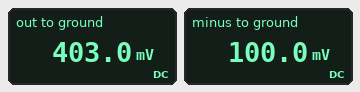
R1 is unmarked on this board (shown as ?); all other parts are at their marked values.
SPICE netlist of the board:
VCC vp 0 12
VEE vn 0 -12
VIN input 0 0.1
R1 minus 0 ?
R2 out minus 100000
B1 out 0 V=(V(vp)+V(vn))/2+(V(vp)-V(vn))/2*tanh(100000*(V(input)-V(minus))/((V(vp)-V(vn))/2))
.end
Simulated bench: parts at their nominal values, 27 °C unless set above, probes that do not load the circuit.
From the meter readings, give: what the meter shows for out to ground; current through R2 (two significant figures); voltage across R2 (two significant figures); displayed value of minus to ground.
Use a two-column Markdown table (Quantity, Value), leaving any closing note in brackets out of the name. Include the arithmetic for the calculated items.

| Quantity | Value |
|---|---|
| what the meter shows for out to ground | 403.0 mV |
| current through R2 | (403 mV - 100 mV) / 100 kΩ = 3.0 µA |
| voltage across R2 | 403 mV - 100 mV = 300 mV |
| displayed value of minus to ground | 100.0 mV |
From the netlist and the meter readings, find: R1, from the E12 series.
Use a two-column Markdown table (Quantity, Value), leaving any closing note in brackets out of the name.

| Quantity | Value |
|---|---|
| R1, from the E12 series | 33 kΩ |
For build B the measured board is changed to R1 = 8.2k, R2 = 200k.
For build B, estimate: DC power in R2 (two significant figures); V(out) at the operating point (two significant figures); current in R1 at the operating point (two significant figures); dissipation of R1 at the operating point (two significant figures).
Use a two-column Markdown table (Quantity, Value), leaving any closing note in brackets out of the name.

| Quantity | Value |
|---|---|
| DC power in R2 | 30 µW |
| V(out) at the operating point | 2.5 V |
| current in R1 at the operating point | 12 µA |
| dissipation of R1 at the operating point | 1.2 µW |
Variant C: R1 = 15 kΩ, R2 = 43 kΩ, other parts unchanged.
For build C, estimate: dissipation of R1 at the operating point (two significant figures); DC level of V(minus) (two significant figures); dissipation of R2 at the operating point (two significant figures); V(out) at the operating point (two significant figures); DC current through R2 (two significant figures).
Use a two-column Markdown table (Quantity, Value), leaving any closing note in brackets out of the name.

| Quantity | Value |
|---|---|
| dissipation of R1 at the operating point | 670 nW |
| DC level of V(minus) | 100 mV |
| dissipation of R2 at the operating point | 1.9 µW |
| V(out) at the operating point | 390 mV |
| DC current through R2 | 6.7 µA |
